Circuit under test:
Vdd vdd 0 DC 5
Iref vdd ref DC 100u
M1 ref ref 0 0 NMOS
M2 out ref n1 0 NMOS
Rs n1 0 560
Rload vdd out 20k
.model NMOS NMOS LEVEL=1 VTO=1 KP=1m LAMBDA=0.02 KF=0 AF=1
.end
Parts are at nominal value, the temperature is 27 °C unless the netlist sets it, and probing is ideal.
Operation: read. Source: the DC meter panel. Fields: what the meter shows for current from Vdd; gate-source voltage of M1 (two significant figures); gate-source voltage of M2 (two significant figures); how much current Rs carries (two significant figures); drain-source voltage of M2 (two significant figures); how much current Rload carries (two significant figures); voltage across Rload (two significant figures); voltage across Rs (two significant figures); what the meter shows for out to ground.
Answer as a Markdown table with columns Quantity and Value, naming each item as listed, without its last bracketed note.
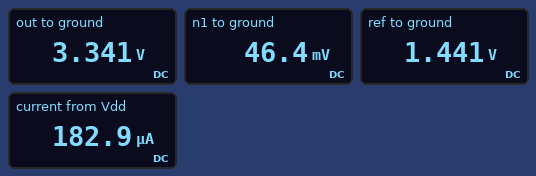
| Quantity | Value |
|---|---|
| what the meter shows for current from Vdd | 182.9 µA |
| gate-source voltage of M1 | 1.4 V |
| gate-source voltage of M2 | 1.4 V |
| how much current Rs carries | 83 µA |
| drain-source voltage of M2 | 3.3 V |
| how much current Rload carries | 83 µA |
| voltage across Rload | 1.7 V |
| voltage across Rs | 46 mV |
| what the meter shows for out to ground | 3.341 V |
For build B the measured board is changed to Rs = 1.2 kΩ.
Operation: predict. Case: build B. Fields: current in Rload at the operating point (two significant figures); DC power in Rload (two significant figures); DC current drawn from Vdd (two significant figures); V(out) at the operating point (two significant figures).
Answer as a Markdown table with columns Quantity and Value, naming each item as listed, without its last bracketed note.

| Quantity | Value |
|---|---|
| current in Rload at the operating point | 69 µA |
| DC power in Rload | 95 µW |
| DC current drawn from Vdd | 170 µA |
| V(out) at the operating point | 3.6 V |
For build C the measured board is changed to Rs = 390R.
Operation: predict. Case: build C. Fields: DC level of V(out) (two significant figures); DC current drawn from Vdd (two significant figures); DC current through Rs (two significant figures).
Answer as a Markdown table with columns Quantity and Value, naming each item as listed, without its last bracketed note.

| Quantity | Value |
|---|---|
| DC level of V(out) | 3.2 V |
| DC current drawn from Vdd | 190 µA |
| DC current through Rs | 88 µA |
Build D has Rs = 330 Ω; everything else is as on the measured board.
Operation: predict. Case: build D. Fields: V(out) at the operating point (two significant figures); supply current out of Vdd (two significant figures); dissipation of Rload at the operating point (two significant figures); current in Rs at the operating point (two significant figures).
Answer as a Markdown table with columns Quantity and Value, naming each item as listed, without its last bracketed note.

| Quantity | Value |
|---|---|
| V(out) at the operating point | 3.2 V |
| supply current out of Vdd | 190 µA |
| dissipation of Rload at the operating point | 160 µW |
| current in Rs at the operating point | 90 µA |
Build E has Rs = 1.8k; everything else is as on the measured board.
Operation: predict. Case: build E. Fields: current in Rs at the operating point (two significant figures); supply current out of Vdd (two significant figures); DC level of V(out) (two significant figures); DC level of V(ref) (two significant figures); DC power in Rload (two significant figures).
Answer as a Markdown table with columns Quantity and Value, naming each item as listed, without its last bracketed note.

| Quantity | Value |
|---|---|
| current in Rs at the operating point | 60 µA |
| supply current out of Vdd | 160 µA |
| DC level of V(out) | 3.8 V |
| DC level of V(ref) | 1.4 V |
| DC power in Rload | 71 µW |
